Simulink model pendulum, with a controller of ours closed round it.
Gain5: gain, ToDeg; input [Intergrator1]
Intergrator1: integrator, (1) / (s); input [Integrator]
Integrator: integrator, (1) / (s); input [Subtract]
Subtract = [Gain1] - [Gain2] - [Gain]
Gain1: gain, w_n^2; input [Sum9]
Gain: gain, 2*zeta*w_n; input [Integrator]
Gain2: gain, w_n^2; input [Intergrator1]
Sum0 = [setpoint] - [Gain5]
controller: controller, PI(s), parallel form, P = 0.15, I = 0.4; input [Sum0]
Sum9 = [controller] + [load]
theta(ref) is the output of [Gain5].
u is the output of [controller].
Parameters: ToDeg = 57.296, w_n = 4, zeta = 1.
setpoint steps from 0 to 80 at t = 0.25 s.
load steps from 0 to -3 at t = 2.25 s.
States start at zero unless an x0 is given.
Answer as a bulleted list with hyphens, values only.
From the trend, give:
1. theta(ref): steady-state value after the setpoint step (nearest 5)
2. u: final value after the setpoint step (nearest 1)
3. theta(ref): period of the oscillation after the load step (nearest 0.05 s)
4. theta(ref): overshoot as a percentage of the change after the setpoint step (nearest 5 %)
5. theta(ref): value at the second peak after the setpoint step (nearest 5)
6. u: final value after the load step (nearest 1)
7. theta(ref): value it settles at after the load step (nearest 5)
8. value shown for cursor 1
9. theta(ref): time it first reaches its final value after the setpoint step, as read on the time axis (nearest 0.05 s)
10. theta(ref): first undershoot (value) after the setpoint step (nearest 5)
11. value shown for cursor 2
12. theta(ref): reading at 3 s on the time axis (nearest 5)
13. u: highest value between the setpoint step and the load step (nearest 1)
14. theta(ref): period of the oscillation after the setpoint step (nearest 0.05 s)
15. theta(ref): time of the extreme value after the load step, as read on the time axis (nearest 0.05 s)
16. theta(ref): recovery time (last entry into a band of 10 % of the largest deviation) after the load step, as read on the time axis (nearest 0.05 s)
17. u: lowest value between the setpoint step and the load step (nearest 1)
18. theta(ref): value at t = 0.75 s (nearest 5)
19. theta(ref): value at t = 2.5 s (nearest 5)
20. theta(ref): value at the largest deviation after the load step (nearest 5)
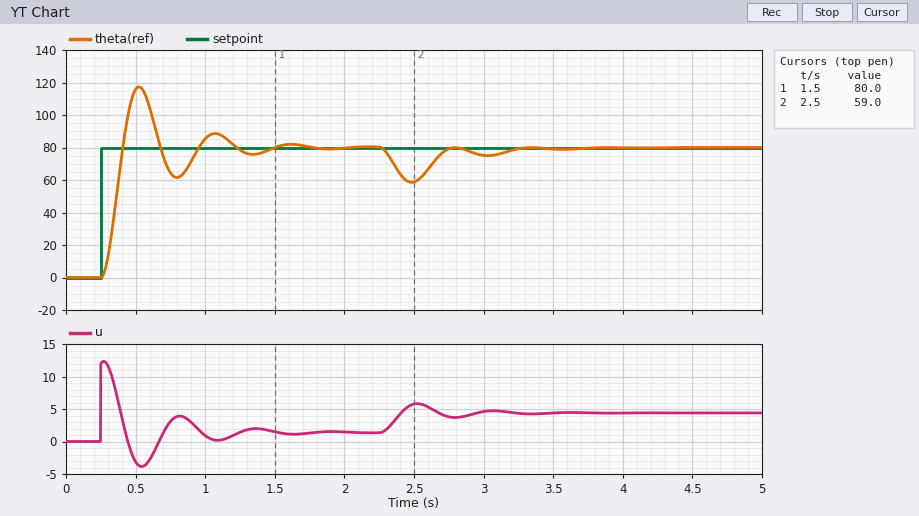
- 80
- 1
- 0.55 s
- 45 %
- 90
- 4
- 80
- 80.0
- 0.40 s
- 60
- 59.0
- 75
- 12
- 0.55 s
- 2.50 s
- 3.20 s
- -4
- 65
- 60
- 60
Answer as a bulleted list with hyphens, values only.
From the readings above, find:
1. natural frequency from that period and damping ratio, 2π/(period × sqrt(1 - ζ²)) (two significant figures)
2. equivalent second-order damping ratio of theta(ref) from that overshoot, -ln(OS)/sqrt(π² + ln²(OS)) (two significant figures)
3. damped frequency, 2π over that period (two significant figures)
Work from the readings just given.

- 12 rad/s
- 0.25
- 11 rad/s
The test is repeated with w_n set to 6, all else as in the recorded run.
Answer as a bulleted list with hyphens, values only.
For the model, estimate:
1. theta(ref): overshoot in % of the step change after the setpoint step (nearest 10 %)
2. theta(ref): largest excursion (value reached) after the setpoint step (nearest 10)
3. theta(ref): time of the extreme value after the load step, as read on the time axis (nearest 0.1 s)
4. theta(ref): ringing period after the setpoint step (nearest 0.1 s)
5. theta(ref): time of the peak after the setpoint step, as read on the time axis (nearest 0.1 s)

- 40 %
- 110
- 2.4 s
- 0.4 s
- 0.4 s
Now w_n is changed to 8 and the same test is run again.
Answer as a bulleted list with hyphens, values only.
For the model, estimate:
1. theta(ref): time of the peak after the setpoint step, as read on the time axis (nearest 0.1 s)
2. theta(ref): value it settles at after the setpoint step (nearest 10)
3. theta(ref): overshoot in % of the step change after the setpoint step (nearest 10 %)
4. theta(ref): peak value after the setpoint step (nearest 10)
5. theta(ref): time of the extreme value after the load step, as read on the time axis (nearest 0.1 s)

- 0.4 s
- 80
- 30 %
- 110
- 2.4 s
